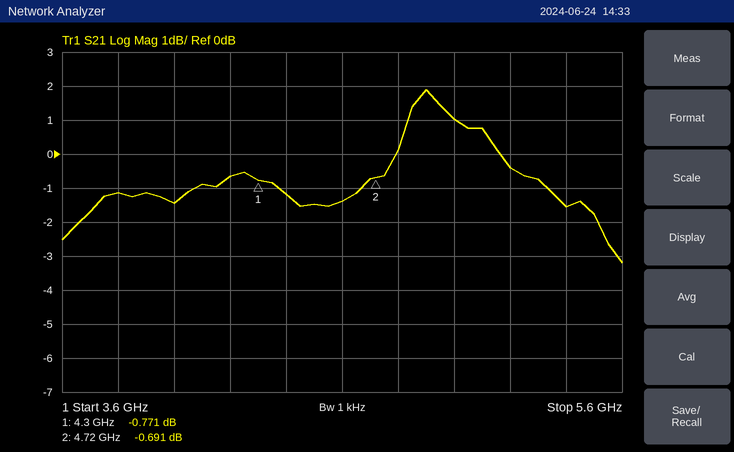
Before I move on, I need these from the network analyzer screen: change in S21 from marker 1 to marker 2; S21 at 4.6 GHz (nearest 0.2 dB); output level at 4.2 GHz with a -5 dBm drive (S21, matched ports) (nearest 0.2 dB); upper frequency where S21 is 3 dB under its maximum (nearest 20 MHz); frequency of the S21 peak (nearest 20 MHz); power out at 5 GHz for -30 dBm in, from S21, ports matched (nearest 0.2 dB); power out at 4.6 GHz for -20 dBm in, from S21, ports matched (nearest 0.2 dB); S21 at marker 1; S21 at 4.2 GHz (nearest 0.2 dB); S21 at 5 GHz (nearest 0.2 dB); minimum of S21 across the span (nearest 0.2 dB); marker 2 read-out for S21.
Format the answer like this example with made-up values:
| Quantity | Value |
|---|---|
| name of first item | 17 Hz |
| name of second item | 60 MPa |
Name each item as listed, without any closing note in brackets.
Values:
| Quantity | Value |
|---|---|
| change in S21 from marker 1 to marker 2 | 0.080 dB |
| S21 at 4.6 GHz | -1.4 dB |
| output level at 4.2 GHz with a -5 dBm drive (S21, matched ports) | -5.6 dBm |
| upper frequency where S21 is 3 dB under its maximum | 5.34 GHz |
| frequency of the S21 peak | 4.90 GHz |
| power out at 5 GHz for -30 dBm in, from S21, ports matched | -29.0 dBm |
| power out at 4.6 GHz for -20 dBm in, from S21, ports matched | -21.4 dBm |
| S21 at marker 1 | -0.771 dB |
| S21 at 4.2 GHz | -0.6 dB |
| S21 at 5 GHz | 1.0 dB |
| minimum of S21 across the span | -3.2 dB |
| marker 2 read-out for S21 | -0.691 dB |
